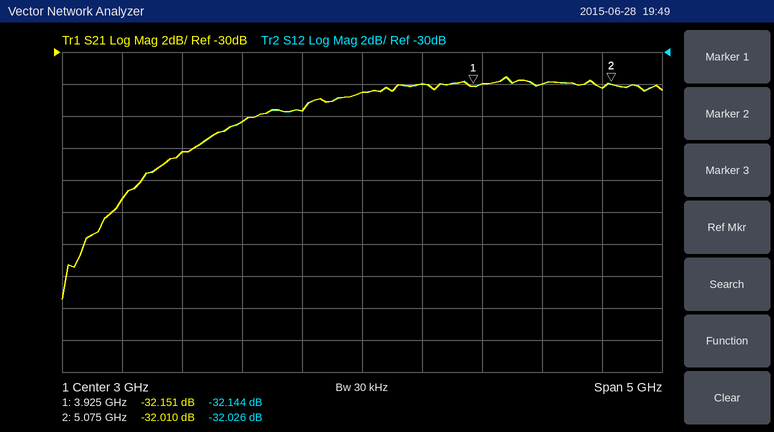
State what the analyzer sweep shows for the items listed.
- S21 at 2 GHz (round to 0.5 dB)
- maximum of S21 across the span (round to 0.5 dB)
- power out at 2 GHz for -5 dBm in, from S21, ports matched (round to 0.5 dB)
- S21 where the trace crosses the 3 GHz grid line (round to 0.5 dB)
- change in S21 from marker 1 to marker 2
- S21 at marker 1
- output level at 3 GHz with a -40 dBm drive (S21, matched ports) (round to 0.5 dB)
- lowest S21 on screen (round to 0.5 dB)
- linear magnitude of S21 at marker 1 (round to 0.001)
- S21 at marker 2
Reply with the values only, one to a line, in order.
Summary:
-34.5 dB
-31.5 dB
-39.5 dBm
-32.5 dB
0.141 dB
-32.151 dB
-72.5 dBm
-45.5 dB
0.025
-32.010 dB
